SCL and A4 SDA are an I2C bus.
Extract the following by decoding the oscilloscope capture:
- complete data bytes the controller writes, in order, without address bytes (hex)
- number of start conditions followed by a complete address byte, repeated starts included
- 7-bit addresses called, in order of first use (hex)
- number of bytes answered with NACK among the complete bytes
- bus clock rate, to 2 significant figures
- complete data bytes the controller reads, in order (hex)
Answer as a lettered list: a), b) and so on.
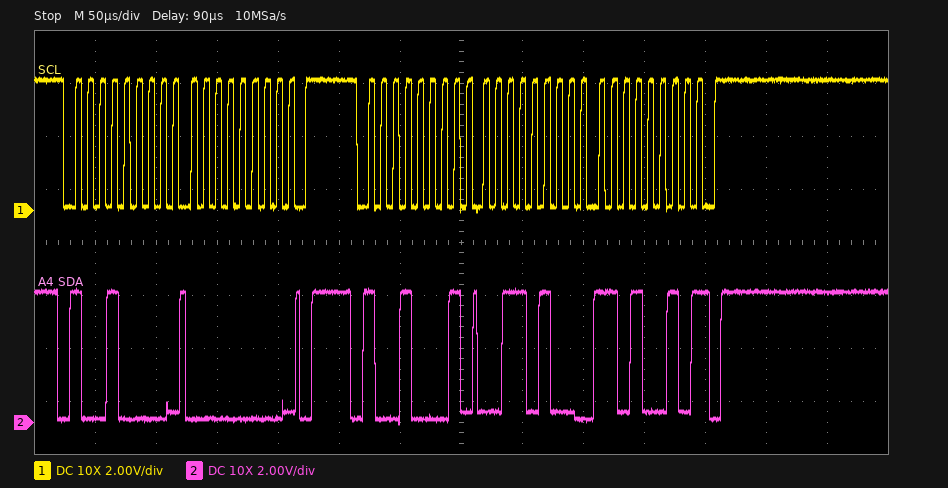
a) 00
b) 2
c) 0x48
d) 1
e) 100 kHz
f) 34 D2
